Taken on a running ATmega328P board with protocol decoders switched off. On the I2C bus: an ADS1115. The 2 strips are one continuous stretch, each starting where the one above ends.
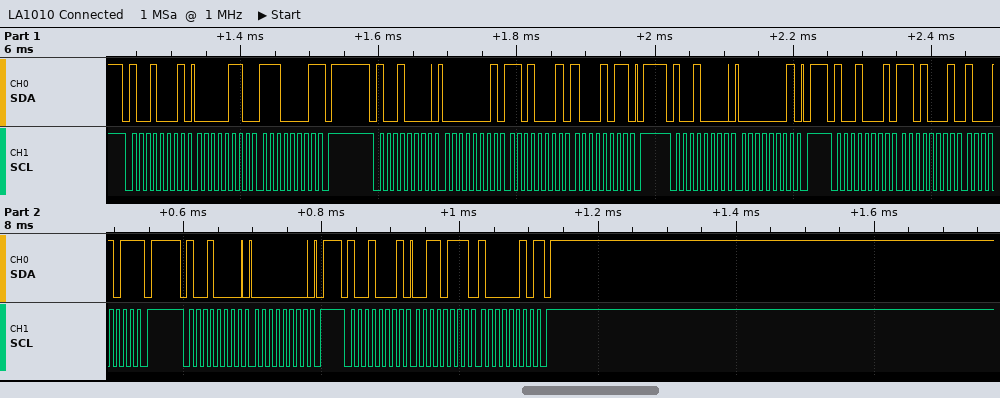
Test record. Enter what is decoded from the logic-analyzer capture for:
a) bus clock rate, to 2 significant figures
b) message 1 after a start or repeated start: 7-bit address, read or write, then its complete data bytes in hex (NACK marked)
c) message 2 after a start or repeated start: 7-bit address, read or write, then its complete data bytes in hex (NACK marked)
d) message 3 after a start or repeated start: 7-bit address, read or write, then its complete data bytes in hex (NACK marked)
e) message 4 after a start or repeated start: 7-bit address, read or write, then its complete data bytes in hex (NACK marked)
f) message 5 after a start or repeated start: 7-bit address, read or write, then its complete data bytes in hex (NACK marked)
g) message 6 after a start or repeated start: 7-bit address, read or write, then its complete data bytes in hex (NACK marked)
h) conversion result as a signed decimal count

100 kHz
0x48 read: 06 E1 NACK
0x48 write: 01 D1 8B
0x48 write: 01
0x48 read: D1 8B NACK
0x48 write: 00
0x48 read: 37 82 NACK
14210
